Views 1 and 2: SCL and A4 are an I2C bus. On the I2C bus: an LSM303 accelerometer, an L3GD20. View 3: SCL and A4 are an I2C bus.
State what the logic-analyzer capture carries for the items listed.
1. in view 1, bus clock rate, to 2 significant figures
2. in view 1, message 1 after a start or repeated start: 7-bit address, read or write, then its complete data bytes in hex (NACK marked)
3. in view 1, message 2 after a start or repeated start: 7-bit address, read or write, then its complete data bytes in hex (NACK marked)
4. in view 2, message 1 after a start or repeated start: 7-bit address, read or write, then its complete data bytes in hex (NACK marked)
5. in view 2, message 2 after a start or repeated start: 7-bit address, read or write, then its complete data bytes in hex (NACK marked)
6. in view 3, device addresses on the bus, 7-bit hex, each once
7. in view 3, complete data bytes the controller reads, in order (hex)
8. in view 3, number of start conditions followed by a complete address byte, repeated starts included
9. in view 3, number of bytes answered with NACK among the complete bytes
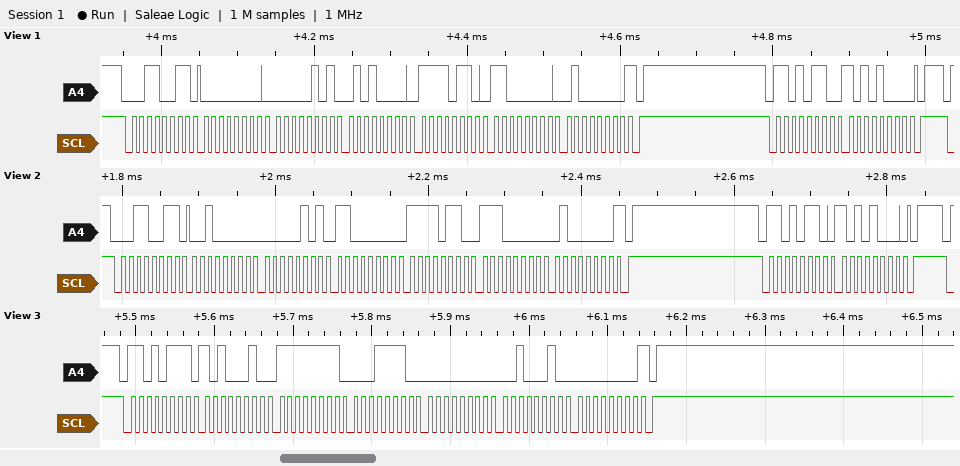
100 kHz
0x19 read: 00 05 50 F6 C0 40 NACK
0x6B write: A8
0x19 read: 20 05 C0 F6 E0 40 NACK
0x6B write: A8
0x6B
A2 FF 1E 00 22 00
1
1
